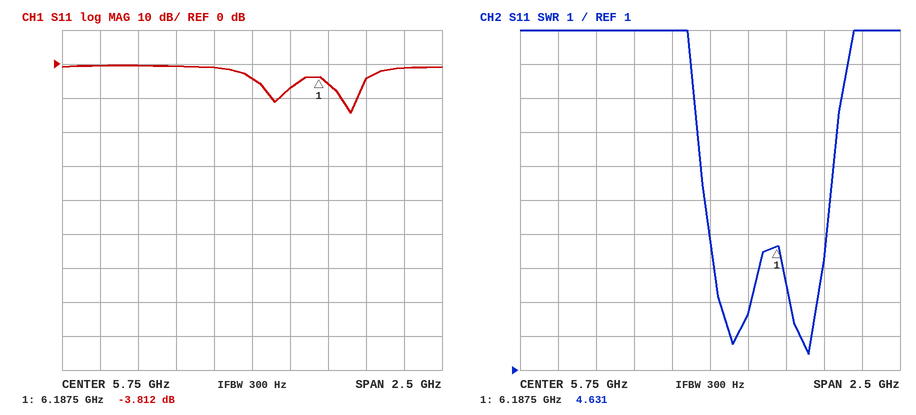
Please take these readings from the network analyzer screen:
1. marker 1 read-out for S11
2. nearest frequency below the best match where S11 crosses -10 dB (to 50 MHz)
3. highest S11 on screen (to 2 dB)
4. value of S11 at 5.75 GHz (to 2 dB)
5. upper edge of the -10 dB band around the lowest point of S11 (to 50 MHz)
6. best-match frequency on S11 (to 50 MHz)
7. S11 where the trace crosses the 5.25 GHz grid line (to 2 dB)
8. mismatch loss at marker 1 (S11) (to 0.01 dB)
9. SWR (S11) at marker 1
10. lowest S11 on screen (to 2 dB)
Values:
-3.812 dB
6.35 GHz
0 dB
-4 dB
6.45 GHz
6.40 GHz
0 dB
2.33 dB
4.631
-14 dB
